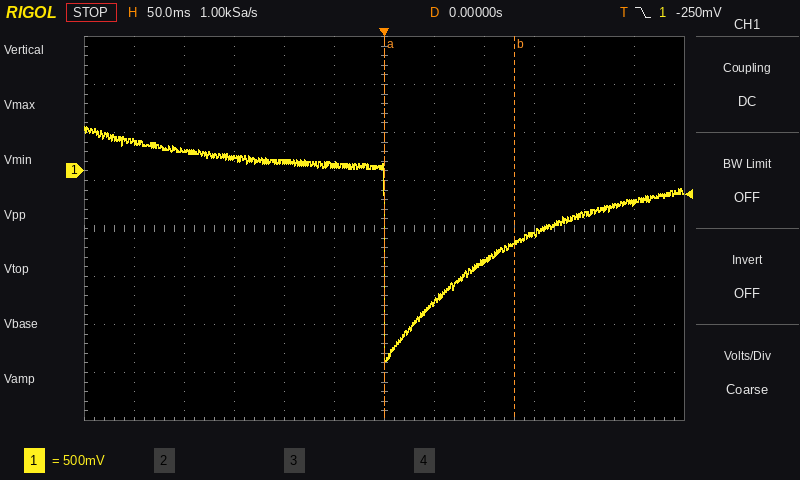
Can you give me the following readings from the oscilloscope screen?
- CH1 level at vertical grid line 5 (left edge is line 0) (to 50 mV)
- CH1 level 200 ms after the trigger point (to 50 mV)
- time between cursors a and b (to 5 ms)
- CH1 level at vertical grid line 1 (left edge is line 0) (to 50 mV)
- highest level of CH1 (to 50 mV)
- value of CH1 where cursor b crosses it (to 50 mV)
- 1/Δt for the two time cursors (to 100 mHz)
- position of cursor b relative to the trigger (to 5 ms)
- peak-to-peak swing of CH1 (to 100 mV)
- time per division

50 mV
-450 mV
130 ms
300 mV
450 mV
-750 mV
7.7 Hz
+130 ms
2.40 V
50 ms
